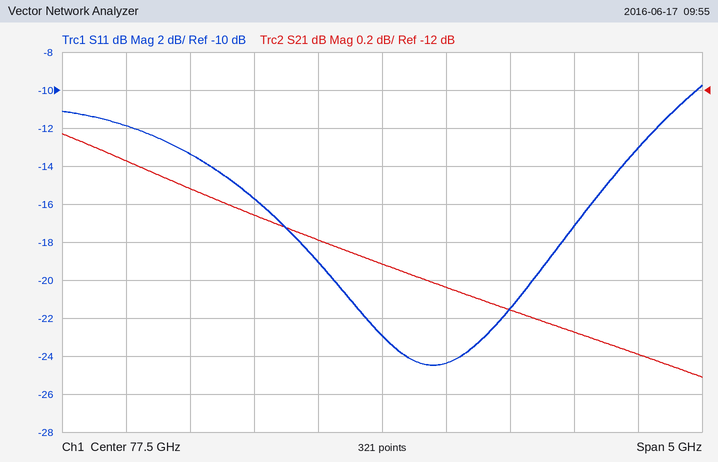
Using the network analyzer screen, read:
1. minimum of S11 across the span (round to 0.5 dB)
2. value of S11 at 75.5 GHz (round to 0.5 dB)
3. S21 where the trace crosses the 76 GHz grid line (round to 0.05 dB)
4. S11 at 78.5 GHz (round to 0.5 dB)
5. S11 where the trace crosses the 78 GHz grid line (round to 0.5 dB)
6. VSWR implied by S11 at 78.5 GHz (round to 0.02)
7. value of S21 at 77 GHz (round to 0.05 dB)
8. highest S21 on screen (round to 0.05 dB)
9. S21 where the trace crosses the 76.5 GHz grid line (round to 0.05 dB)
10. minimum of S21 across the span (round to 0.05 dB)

-24.5 dB
-12.0 dB
-12.50 dB
-21.5 dB
-24.5 dB
1.18
-12.80 dB
-12.25 dB
-12.65 dB
-13.50 dB
